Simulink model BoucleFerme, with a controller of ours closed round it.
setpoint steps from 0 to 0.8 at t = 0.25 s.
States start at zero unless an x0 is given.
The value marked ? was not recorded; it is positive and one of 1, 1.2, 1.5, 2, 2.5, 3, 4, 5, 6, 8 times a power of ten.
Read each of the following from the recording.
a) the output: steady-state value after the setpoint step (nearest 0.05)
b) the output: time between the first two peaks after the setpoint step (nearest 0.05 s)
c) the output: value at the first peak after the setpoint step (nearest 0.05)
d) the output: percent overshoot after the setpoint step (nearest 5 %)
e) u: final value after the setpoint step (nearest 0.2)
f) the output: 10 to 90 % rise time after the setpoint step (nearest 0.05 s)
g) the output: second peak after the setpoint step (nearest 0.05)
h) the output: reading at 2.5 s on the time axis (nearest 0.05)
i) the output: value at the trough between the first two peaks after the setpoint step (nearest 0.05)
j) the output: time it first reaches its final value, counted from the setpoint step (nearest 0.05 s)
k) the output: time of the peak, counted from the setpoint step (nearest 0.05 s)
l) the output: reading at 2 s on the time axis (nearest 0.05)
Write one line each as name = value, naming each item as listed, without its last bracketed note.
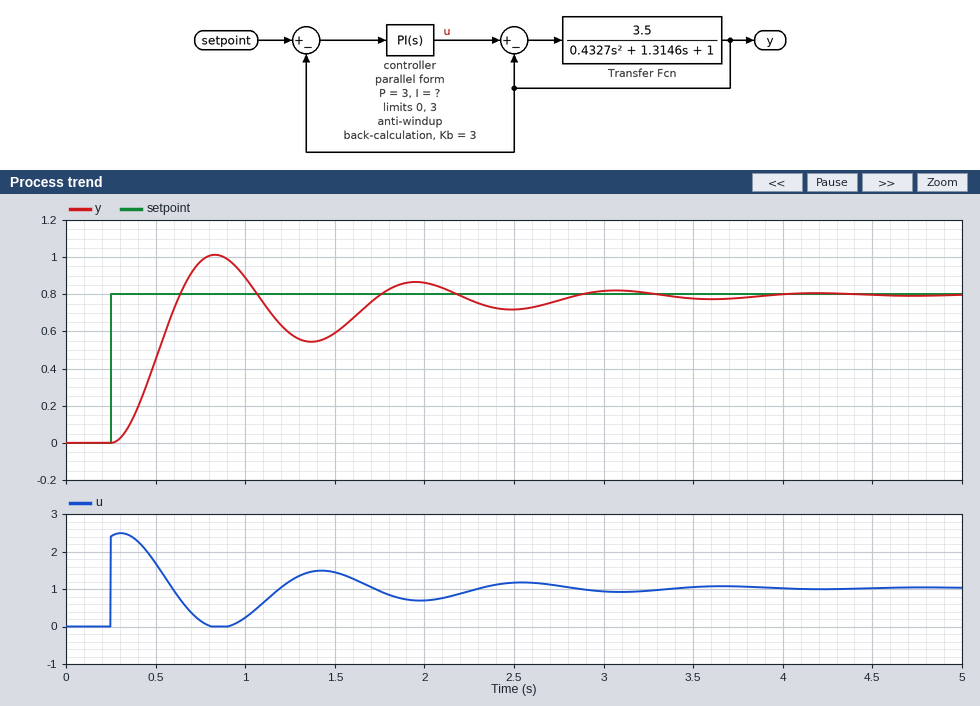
the output: steady-state value after the setpoint step = 0.80
the output: time between the first two peaks after the setpoint step = 1.10 s
the output: value at the first peak after the setpoint step = 1.00
the output: percent overshoot after the setpoint step = 25 %
u: final value after the setpoint step = 1.0
the output: 10 to 90 % rise time after the setpoint step = 0.25 s
the output: second peak after the setpoint step = 0.85
the output: reading at 2.5 s on the time axis = 0.70
the output: value at the trough between the first two peaks after the setpoint step = 0.55
the output: time it first reaches its final value, counted from the setpoint step = 0.40 s
the output: time of the peak, counted from the setpoint step = 0.60 s
the output: reading at 2 s on the time axis = 0.85
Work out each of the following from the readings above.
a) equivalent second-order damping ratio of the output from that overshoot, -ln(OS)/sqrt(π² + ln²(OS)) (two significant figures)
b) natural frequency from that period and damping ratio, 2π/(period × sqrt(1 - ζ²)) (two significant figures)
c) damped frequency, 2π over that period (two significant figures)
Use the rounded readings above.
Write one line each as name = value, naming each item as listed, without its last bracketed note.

equivalent second-order damping ratio of the output from that overshoot, -ln(OS)/sqrt(π² + ln²(OS)) = 0.40
natural frequency from that period and damping ratio, 2π/(period × sqrt(1 - ζ²)) = 6.2 rad/s
damped frequency, 2π over that period = 5.7 rad/s
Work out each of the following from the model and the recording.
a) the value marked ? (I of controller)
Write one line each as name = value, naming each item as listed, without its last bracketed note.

the value marked ? = 4
